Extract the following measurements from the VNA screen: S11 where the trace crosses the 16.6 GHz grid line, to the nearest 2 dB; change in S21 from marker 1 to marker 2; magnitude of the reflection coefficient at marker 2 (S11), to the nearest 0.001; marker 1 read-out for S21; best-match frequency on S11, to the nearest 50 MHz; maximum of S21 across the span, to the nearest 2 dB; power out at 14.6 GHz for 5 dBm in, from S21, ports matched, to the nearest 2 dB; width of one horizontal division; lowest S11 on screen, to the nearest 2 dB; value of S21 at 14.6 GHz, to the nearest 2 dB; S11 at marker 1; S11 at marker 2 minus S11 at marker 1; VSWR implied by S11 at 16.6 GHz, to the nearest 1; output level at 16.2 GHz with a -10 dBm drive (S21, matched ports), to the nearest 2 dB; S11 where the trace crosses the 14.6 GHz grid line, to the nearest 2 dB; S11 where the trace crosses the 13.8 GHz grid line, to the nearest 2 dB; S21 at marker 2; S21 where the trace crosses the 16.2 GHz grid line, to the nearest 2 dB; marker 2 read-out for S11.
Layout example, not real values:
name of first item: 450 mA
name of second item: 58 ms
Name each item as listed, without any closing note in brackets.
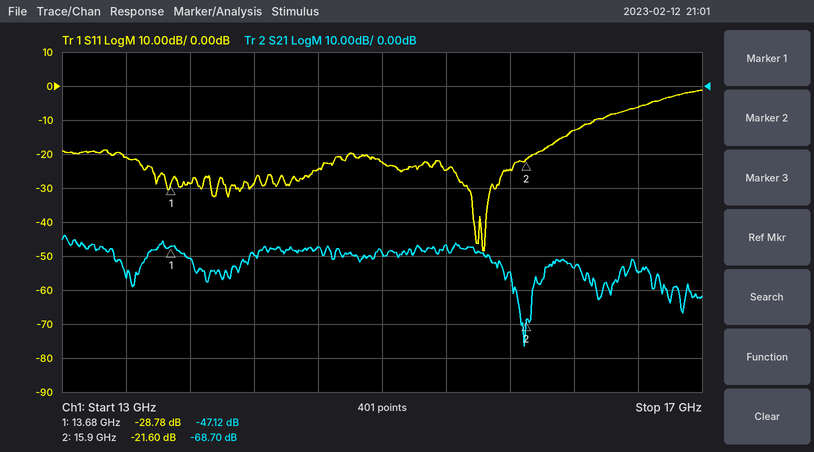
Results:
S11 where the trace crosses the 16.6 GHz grid line, to the nearest 2 dB: -6 dB
change in S21 from marker 1 to marker 2: -21.58 dB
magnitude of the reflection coefficient at marker 2 (S11), to the nearest 0.001: 0.083
marker 1 read-out for S21: -47.12 dB
best-match frequency on S11, to the nearest 50 MHz: 15.65 GHz
maximum of S21 across the span, to the nearest 2 dB: -44 dB
power out at 14.6 GHz for 5 dBm in, from S21, ports matched, to the nearest 2 dB: -42 dBm
width of one horizontal division: 400 MHz
lowest S11 on screen, to the nearest 2 dB: -48 dB
value of S21 at 14.6 GHz, to the nearest 2 dB: -48 dB
S11 at marker 1: -28.78 dB
S11 at marker 2 minus S11 at marker 1: 7.18 dB
VSWR implied by S11 at 16.6 GHz, to the nearest 1: 3
output level at 16.2 GHz with a -10 dBm drive (S21, matched ports), to the nearest 2 dB: -64 dBm
S11 where the trace crosses the 14.6 GHz grid line, to the nearest 2 dB: -24 dB
S11 where the trace crosses the 13.8 GHz grid line, to the nearest 2 dB: -28 dB
S21 at marker 2: -68.70 dB
S21 where the trace crosses the 16.2 GHz grid line, to the nearest 2 dB: -54 dB
marker 2 read-out for S11: -21.60 dB
